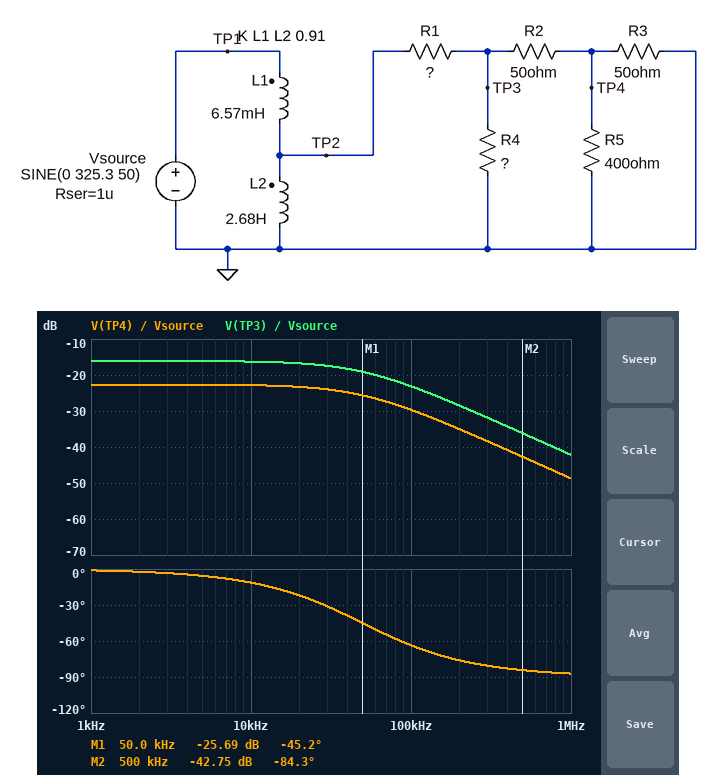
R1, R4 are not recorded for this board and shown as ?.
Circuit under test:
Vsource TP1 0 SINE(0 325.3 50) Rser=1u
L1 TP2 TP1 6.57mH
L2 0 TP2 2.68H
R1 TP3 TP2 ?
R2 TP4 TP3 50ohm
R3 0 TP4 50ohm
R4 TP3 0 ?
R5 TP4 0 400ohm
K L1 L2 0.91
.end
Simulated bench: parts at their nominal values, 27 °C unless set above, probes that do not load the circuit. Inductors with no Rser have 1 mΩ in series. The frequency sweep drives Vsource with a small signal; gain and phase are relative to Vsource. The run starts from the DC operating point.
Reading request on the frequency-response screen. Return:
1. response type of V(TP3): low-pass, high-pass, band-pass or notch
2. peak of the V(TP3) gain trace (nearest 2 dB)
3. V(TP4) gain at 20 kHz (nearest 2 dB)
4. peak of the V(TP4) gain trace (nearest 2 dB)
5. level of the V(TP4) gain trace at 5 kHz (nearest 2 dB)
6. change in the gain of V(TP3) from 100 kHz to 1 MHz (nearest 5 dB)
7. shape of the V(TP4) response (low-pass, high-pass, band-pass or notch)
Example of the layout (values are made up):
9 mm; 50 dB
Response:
low-pass; -16 dB; -24 dB; -22 dB; -22 dB; -20 dB; low-pass
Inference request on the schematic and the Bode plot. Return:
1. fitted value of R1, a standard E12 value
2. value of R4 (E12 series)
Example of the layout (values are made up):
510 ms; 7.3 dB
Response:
270 Ω; 120 Ω
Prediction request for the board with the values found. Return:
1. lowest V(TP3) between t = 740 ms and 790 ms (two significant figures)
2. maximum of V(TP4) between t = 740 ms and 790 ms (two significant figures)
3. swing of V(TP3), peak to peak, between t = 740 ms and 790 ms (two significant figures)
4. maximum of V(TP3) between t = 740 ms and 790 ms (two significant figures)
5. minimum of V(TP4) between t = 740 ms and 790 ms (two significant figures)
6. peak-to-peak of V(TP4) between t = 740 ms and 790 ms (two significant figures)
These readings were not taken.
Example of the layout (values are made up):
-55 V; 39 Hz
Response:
-51 V; 24 V; 100 V; 51 V; -24 V; 48 V
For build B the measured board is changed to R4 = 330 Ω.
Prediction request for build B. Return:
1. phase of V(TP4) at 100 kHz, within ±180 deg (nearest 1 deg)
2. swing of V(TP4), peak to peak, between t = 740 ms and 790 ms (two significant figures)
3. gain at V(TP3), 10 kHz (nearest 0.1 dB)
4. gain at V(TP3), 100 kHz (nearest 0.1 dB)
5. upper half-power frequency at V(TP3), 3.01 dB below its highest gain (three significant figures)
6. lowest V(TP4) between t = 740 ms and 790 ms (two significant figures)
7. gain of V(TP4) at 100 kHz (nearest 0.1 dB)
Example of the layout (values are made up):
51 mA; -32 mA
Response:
-62 deg; 63 V; -13.9 dB; -20.4 dB; 52.9 kHz; -31 V; -26.9 dB
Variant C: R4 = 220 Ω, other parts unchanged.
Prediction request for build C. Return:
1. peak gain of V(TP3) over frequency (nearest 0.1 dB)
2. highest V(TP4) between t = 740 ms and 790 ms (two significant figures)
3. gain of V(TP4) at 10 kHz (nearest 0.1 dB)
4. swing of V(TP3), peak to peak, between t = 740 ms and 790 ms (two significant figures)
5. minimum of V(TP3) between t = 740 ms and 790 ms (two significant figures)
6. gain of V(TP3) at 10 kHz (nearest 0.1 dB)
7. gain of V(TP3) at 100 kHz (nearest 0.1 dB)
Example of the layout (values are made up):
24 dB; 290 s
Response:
-14.5 dB; 29 V; -21.2 dB; 120 V; -61 V; -14.7 dB; -21.3 dB
